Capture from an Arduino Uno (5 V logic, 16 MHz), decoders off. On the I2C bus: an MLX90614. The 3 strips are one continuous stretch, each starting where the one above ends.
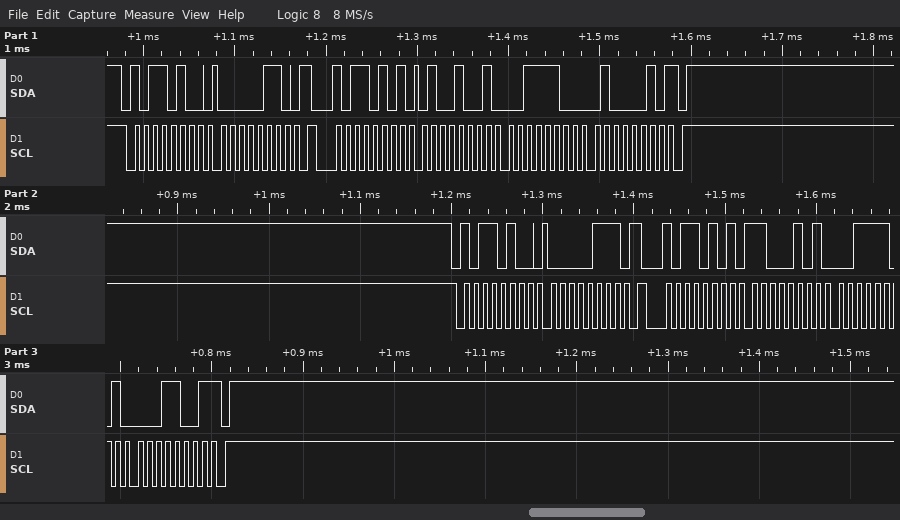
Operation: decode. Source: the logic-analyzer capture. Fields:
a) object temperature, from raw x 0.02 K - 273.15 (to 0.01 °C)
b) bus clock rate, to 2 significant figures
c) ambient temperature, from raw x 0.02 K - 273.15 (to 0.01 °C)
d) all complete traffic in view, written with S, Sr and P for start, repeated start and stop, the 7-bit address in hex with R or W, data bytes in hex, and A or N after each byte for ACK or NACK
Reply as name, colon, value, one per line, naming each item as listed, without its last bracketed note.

object temperature, from raw x 0.02 K - 273.15: 43.11 °C
bus clock rate, to 2 significant figures: 100 kHz
ambient temperature, from raw x 0.02 K - 273.15: 35.51 °C
all complete traffic in view, written with S, Sr and P for start, repeated start and stop, the 7-bit address in hex with R or W, data bytes in hex, and A or N after each byte for ACK or NACK: S 5AW A 06 A Sr 5AR A 49 A 3C A 42 N P S 5AW A 07 A Sr 5AR A C5 A 3D A 19 N P
